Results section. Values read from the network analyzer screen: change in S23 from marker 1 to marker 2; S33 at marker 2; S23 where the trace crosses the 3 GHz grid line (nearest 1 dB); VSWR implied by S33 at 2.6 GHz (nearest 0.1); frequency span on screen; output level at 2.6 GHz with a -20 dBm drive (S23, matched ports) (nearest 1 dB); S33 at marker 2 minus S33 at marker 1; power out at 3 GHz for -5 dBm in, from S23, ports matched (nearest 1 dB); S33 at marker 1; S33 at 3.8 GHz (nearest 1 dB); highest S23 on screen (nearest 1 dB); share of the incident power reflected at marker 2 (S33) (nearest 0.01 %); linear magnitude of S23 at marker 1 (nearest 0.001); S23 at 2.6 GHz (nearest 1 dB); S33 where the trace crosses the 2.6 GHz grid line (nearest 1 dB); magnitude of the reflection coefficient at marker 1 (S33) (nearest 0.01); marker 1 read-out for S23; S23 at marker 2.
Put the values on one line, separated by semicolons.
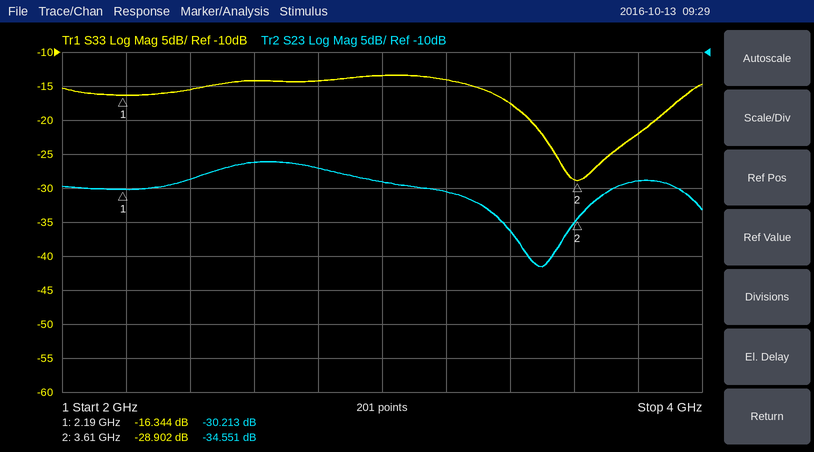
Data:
-4.338 dB; -28.902 dB; -29 dB; 1.5; 2 GHz; -46 dBm; -12.558 dB; -34 dBm; -16.344 dB; -22 dB; -26 dB; 0.13 %; 0.031; -26 dB; -14 dB; 0.15; -30.213 dB; -34.551 dB
